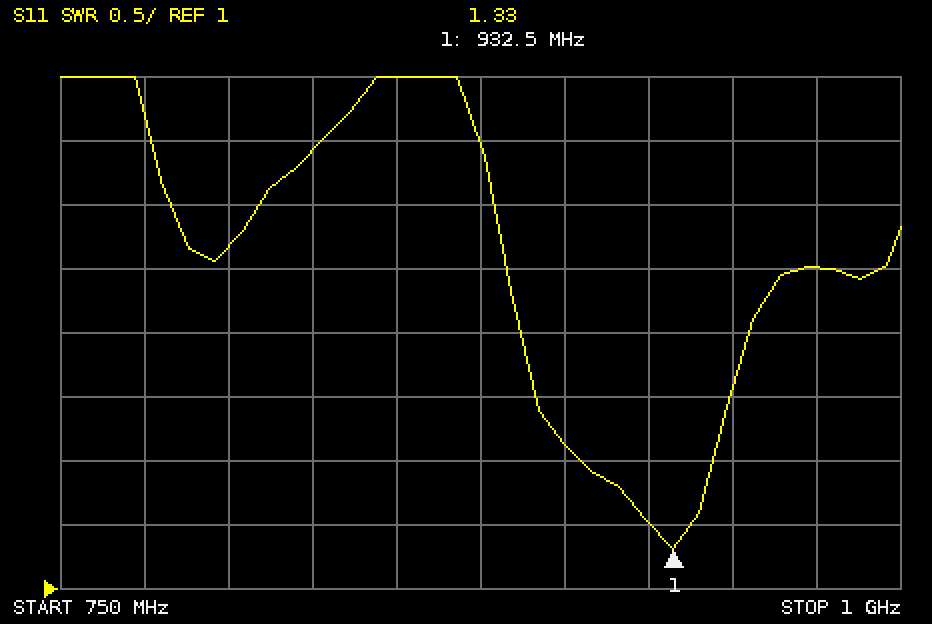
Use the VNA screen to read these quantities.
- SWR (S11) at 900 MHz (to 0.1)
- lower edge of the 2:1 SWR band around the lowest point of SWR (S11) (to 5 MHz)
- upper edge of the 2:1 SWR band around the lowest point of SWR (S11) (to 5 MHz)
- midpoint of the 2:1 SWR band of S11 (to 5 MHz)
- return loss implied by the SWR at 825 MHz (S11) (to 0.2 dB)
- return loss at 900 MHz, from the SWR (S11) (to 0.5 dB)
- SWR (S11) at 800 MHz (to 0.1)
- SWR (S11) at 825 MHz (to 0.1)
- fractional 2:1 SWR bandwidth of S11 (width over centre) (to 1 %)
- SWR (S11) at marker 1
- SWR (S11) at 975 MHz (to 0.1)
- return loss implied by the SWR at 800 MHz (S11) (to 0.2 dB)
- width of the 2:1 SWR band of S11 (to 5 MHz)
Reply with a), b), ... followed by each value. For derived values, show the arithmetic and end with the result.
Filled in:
a) 2.1
b) 905 MHz
c) 945 MHz
d) 925 MHz
e) −20 log10((4.4 − 1)/(4.4 + 1)) ≈ 4.0 dB
f) −20 log10((2.1 − 1)/(2.1 + 1)) ≈ 9.0 dB
g) 3.7
h) 4.4
i) 40 MHz / 925 MHz ≈ 4 %
j) 1.33
k) 3.5
l) −20 log10((3.7 − 1)/(3.7 + 1)) ≈ 4.8 dB
m) 945 MHz − 905 MHz = 40 MHz
